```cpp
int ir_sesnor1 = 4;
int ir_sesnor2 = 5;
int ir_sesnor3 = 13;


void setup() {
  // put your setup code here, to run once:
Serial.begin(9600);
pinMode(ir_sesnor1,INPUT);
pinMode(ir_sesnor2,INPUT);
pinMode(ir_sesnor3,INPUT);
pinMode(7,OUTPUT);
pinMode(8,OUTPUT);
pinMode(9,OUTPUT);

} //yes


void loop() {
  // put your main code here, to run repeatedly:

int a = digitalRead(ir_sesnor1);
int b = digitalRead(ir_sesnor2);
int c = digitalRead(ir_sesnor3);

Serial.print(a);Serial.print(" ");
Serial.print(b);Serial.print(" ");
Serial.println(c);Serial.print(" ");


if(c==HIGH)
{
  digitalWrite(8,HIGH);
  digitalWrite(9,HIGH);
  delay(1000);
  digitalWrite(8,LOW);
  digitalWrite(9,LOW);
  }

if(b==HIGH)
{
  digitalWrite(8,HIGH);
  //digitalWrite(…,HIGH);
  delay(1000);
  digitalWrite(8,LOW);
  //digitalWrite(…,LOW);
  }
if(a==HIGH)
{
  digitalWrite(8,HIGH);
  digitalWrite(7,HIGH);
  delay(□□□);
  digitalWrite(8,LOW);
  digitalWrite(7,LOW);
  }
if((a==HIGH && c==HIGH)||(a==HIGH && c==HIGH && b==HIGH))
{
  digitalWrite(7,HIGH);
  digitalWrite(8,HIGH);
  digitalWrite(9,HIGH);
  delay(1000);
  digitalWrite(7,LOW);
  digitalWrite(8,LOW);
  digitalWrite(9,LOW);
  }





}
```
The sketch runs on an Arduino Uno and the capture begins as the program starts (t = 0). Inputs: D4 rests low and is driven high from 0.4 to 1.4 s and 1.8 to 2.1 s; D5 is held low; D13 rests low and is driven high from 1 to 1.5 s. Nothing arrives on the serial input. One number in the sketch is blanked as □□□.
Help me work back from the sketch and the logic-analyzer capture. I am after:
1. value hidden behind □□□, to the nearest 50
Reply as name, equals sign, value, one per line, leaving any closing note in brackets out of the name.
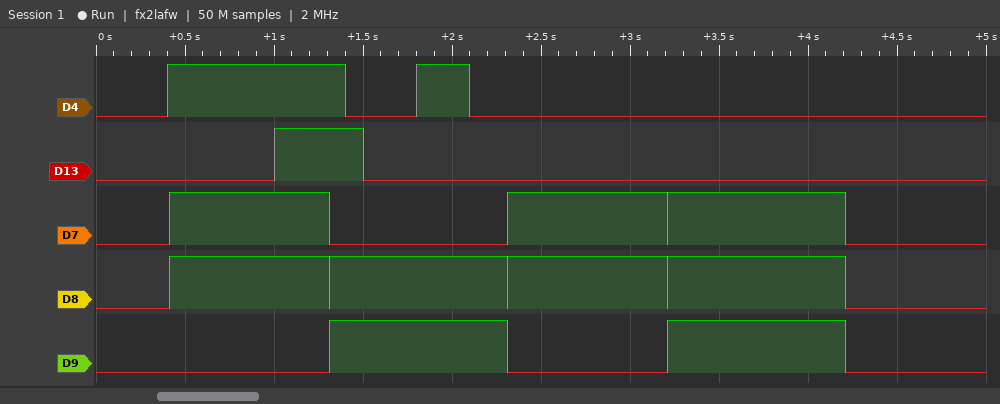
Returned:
value hidden behind □□□, to the nearest 50 = 900
